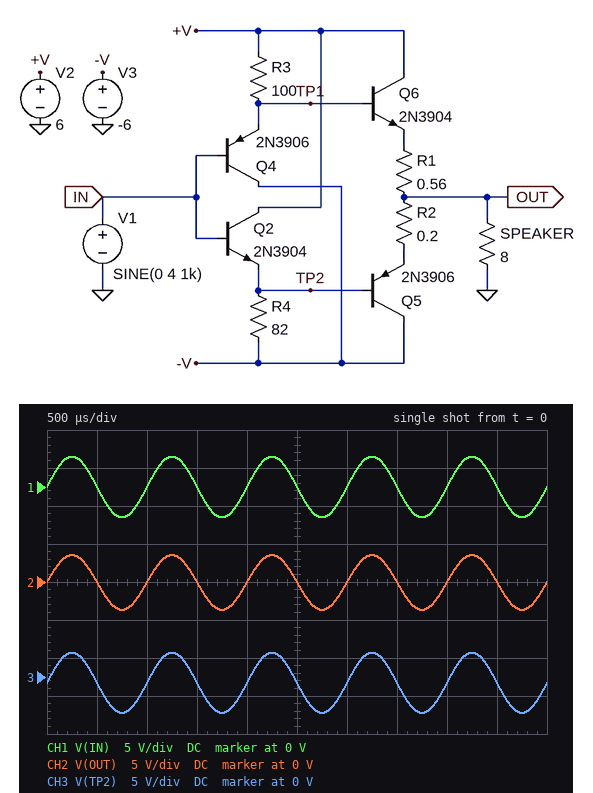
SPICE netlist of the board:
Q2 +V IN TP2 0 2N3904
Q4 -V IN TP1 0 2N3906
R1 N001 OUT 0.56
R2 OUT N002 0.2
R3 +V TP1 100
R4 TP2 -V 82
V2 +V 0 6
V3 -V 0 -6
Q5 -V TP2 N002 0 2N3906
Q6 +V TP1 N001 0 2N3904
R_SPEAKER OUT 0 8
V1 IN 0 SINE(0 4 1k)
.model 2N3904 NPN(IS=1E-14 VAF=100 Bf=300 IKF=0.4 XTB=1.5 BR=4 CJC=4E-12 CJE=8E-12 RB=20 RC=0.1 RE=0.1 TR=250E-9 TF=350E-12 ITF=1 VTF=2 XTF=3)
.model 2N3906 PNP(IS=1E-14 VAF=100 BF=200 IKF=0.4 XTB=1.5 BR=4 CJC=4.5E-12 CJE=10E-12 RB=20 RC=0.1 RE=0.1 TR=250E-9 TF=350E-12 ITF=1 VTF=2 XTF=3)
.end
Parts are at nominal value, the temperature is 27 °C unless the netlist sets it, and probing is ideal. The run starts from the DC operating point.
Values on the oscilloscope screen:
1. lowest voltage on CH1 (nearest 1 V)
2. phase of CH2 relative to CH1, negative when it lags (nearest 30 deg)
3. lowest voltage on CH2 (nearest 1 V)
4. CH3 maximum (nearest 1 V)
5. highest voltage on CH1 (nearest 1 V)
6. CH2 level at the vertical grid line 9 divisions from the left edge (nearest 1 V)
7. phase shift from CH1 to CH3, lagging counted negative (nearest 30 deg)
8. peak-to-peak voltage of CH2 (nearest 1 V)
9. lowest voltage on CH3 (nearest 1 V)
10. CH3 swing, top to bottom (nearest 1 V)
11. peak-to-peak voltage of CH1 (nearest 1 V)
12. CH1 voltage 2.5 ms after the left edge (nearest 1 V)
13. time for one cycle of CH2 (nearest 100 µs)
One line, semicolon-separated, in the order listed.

-4 V; 0 deg; -4 V; 3 V; 4 V; 0 V; 0 deg; 7 V; -5 V; 8 V; 8 V; 0 V; 1.0 ms
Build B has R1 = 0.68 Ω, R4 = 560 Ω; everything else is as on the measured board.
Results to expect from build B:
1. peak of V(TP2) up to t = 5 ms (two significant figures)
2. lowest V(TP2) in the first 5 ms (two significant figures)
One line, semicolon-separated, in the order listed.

3.3 V; -4.0 V
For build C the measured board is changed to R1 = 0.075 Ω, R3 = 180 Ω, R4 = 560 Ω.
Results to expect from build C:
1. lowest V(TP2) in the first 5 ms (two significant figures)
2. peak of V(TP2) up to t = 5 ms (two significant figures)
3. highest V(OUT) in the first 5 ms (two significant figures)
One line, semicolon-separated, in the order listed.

-4.0 V; 3.3 V; 3.7 V
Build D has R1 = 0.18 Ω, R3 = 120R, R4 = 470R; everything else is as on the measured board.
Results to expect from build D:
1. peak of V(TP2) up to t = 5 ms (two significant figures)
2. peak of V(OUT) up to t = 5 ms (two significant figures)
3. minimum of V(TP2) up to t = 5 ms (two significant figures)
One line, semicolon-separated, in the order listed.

3.3 V; 3.7 V; -4.2 V
